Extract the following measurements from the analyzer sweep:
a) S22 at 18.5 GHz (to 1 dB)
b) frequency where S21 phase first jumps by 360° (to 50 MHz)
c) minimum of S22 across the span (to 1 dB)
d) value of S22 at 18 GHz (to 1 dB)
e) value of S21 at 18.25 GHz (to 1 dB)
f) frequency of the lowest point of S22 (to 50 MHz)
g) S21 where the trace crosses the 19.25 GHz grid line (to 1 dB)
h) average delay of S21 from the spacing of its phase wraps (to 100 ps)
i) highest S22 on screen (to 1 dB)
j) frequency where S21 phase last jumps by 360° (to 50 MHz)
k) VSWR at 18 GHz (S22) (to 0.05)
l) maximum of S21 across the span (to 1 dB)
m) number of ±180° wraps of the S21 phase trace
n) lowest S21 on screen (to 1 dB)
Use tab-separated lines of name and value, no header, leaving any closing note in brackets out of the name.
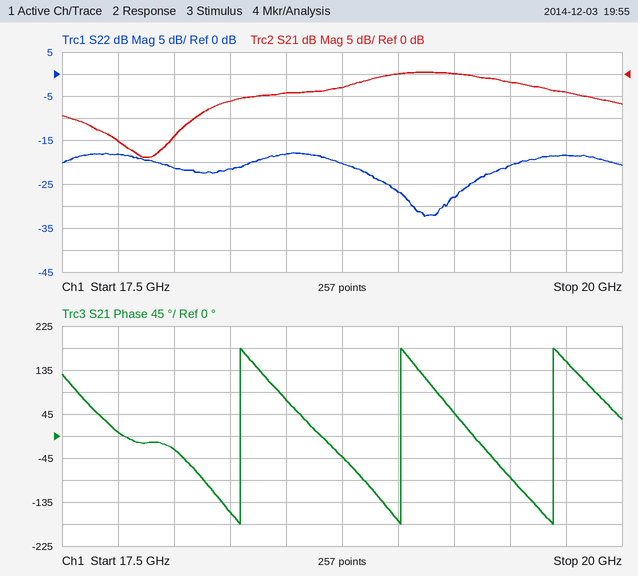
S22 at 18.5 GHz	-18 dB
frequency where S21 phase first jumps by 360°	18.30 GHz
minimum of S22 across the span	-32 dB
value of S22 at 18 GHz	-21 dB
value of S21 at 18.25 GHz	-6 dB
frequency of the lowest point of S22	19.10 GHz
S21 where the trace crosses the 19.25 GHz grid line	0 dB
average delay of S21 from the spacing of its phase wraps	1.4 ns
highest S22 on screen	-18 dB
frequency where S21 phase last jumps by 360°	19.70 GHz
VSWR at 18 GHz (S22)	1.20
maximum of S21 across the span	0 dB
number of ±180° wraps of the S21 phase trace	3
lowest S21 on screen	-19 dB
